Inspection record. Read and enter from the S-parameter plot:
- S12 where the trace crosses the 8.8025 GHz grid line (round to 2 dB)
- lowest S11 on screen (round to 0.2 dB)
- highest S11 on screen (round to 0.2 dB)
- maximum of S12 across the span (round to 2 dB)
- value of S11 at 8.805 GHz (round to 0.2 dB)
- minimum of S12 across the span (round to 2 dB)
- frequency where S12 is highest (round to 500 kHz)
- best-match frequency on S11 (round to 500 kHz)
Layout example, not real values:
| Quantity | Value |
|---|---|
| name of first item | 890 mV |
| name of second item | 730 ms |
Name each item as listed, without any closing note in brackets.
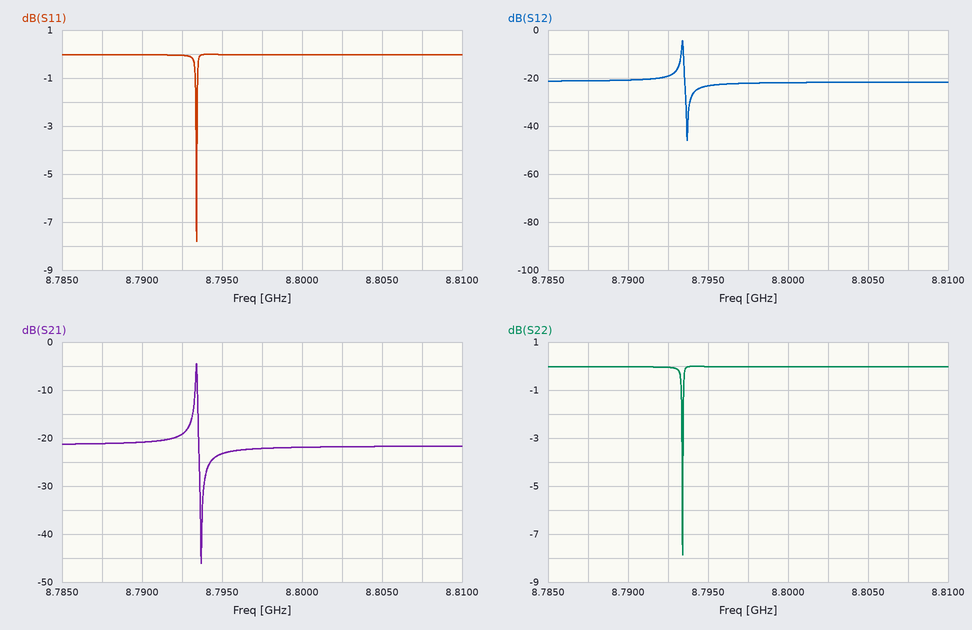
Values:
| Quantity | Value |
|---|---|
| S12 where the trace crosses the 8.8025 GHz grid line | -22 dB |
| lowest S11 on screen | -7.8 dB |
| highest S11 on screen | 0.0 dB |
| maximum of S12 across the span | -4 dB |
| value of S11 at 8.805 GHz | 0.0 dB |
| minimum of S12 across the span | -46 dB |
| frequency where S12 is highest | 8.7935 GHz |
| best-match frequency on S11 | 8.7935 GHz |
